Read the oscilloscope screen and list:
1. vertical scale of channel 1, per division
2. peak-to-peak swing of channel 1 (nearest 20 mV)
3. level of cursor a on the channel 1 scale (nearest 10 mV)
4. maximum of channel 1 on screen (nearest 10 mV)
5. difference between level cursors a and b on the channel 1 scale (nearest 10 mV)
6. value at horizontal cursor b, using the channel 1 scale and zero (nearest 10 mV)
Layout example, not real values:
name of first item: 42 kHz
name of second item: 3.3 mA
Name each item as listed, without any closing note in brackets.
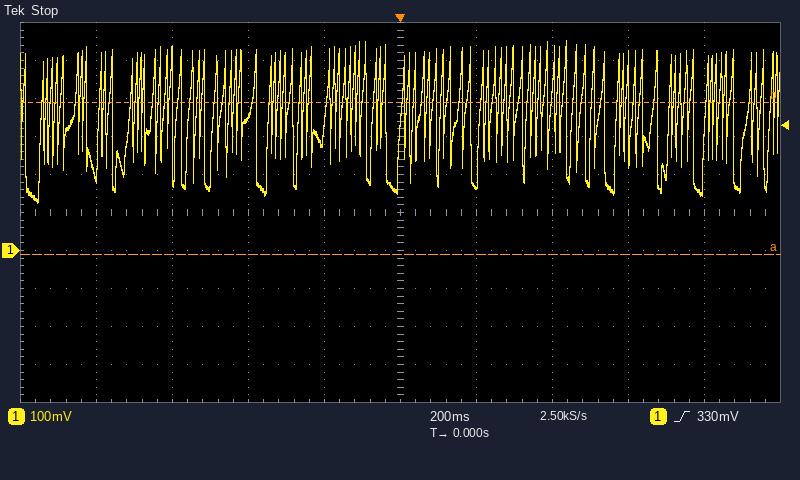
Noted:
vertical scale of channel 1, per division: 100 mV
peak-to-peak swing of channel 1: 420 mV
level of cursor a on the channel 1 scale: -10 mV
maximum of channel 1 on screen: 550 mV
difference between level cursors a and b on the channel 1 scale: 400 mV
value at horizontal cursor b, using the channel 1 scale and zero: 390 mV
